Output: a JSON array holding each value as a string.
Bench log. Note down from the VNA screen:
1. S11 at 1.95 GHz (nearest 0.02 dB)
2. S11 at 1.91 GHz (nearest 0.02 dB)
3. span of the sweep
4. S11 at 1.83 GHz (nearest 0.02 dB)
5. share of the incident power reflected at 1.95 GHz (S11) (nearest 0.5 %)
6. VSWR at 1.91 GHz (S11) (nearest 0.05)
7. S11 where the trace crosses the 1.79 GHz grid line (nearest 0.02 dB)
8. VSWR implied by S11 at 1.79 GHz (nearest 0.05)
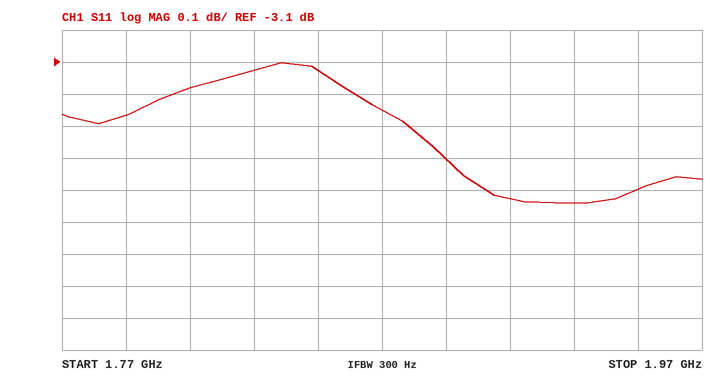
["-3.50 dB", "-3.52 dB", "200 MHz", "-3.12 dB", "44.5 %", "5.00", "-3.26 dB", "5.40"]
